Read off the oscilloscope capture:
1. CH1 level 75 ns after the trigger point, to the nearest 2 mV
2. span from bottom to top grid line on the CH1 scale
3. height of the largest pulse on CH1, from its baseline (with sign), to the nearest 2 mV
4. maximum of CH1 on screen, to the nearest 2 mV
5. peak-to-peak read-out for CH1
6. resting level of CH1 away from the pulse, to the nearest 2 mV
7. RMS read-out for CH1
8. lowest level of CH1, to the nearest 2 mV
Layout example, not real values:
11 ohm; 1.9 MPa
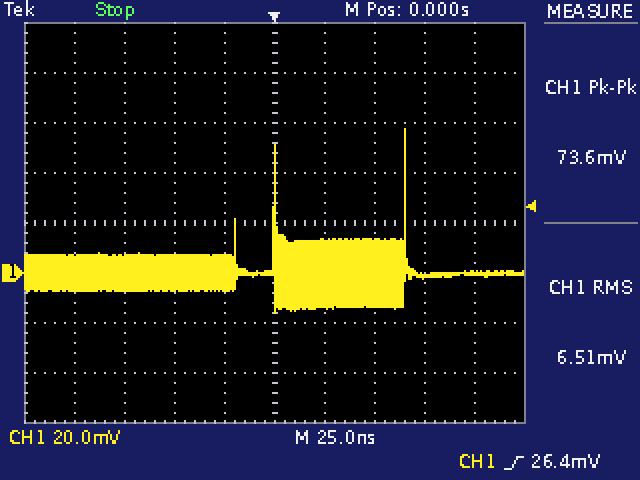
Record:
-2 mV; 160 mV; +58 mV; 58 mV; 73.6 mV; 0 mV; 6.51 mV; -16 mV
